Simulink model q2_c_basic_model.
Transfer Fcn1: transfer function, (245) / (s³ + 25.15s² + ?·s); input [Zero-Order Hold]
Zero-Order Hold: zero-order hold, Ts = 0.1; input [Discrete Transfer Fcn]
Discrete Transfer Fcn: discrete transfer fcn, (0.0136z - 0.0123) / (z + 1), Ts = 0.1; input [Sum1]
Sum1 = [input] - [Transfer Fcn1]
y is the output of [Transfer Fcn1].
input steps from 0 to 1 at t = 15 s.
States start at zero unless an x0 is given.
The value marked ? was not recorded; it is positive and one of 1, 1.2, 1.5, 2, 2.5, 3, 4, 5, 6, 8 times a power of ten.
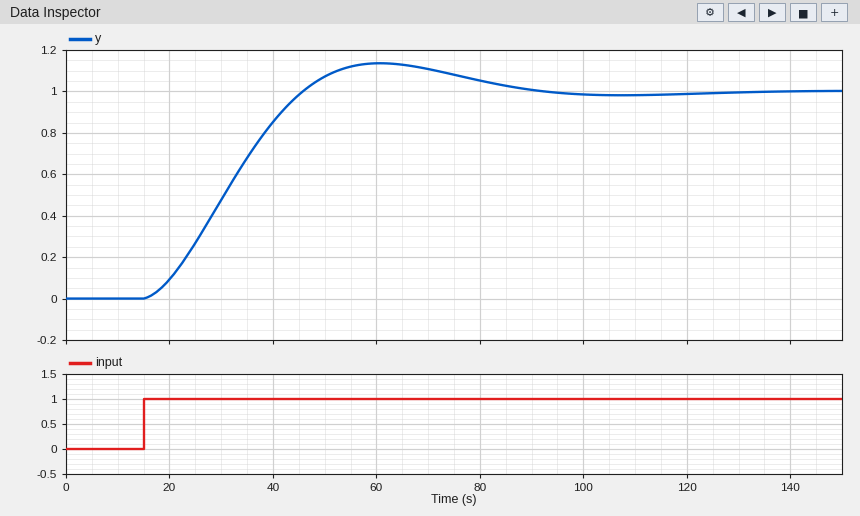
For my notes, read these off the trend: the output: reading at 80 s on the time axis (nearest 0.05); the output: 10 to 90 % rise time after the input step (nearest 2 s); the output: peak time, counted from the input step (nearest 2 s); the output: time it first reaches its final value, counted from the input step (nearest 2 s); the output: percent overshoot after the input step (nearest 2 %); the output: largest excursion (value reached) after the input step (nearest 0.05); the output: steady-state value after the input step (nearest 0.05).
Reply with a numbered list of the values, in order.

1. 1.05
2. 22 s
3. 46 s
4. 30 s
5. 14 %
6. 1.15
7. 1.00
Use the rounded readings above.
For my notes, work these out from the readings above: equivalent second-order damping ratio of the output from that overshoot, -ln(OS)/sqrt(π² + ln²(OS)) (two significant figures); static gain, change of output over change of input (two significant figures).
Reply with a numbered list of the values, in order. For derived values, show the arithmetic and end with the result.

1. ln(0.14) = -1.966; 1.966 / sqrt(9.870 + 3.866) = 0.53
2. (1 - 0) / (1 - 0) = 1.0
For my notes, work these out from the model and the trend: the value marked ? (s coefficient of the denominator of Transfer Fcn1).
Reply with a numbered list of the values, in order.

1. 2
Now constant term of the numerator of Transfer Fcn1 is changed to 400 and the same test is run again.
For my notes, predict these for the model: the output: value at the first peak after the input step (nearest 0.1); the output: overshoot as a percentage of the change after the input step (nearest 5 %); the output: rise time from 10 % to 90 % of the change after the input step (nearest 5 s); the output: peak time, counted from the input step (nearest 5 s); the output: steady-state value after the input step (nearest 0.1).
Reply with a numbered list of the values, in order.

1. 1.2
2. 20 %
3. 15 s
4. 35 s
5. 1.0
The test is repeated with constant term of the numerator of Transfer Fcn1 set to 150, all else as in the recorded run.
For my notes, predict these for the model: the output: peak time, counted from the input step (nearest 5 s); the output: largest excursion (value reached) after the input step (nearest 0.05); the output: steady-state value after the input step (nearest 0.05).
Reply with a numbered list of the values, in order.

1. 65 s
2. 1.05
3. 1.00
